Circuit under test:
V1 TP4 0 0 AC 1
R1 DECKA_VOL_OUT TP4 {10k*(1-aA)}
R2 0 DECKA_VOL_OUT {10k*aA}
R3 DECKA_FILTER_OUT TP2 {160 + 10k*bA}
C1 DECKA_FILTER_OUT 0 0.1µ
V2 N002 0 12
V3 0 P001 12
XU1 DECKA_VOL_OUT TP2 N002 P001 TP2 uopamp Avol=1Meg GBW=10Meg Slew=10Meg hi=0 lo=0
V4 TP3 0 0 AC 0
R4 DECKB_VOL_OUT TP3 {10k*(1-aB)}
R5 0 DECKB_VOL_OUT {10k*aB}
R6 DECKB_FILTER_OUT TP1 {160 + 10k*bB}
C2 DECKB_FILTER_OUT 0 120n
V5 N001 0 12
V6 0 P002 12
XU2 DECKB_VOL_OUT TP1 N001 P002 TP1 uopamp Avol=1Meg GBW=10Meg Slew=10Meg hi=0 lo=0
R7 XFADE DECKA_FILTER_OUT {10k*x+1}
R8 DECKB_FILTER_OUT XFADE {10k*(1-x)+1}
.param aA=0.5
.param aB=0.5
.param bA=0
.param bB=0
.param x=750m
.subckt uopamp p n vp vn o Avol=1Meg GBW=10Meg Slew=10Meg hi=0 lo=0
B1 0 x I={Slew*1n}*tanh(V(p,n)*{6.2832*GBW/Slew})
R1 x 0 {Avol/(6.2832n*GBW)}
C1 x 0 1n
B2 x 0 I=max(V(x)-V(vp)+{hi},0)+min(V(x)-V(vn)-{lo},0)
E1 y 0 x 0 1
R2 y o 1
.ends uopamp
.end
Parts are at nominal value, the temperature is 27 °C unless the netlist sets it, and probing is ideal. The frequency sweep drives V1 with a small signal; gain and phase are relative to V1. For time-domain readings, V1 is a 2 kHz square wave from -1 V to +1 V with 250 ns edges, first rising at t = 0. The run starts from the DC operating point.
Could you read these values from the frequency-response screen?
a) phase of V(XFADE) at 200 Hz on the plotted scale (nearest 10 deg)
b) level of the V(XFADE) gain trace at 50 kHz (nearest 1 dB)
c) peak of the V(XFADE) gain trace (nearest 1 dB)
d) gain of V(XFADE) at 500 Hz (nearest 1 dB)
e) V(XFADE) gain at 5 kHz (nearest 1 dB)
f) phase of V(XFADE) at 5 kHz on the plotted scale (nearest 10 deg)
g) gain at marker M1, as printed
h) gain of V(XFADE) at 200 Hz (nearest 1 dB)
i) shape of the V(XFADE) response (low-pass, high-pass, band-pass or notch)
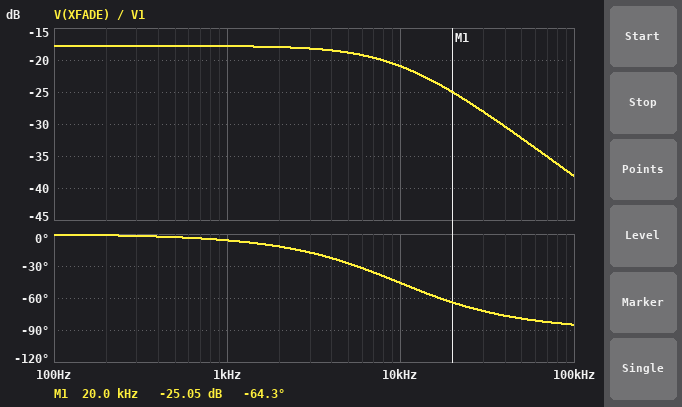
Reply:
0 deg
-32 dB
-18 dB
-18 dB
-19 dB
-30 deg
-25.05 dB
-18 dB
low-pass
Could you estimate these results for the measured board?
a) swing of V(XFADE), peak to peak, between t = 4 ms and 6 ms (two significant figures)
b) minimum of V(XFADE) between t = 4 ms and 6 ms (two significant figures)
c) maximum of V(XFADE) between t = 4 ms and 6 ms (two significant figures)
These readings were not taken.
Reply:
260 mV
-130 mV
130 mV
